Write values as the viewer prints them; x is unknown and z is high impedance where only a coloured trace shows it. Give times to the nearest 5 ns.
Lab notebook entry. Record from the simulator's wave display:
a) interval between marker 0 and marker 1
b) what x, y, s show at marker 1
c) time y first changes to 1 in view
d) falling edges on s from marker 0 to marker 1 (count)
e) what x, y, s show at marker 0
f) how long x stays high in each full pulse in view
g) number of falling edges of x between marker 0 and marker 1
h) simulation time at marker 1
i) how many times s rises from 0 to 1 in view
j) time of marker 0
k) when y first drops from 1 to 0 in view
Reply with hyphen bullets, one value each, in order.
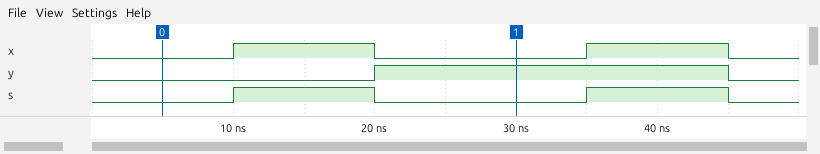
- 25 ns
- x=0, y=1, s=0
- 20 ns
- 1
- x=0, y=0, s=0
- 10 ns, 10 ns
- 1
- 30 ns
- 2
- 5 ns
- 45 ns
